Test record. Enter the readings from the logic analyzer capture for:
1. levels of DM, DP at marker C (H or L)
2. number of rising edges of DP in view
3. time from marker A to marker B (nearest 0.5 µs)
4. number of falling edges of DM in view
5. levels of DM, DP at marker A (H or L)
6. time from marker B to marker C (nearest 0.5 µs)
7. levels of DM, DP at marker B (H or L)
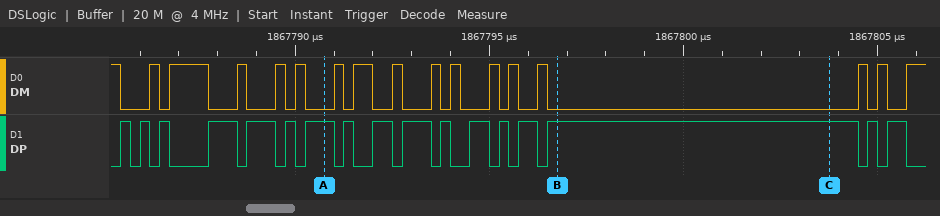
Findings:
DM=L, DP=H
17
6 µs
16
DM=L, DP=H
7 µs
DM=L, DP=H
